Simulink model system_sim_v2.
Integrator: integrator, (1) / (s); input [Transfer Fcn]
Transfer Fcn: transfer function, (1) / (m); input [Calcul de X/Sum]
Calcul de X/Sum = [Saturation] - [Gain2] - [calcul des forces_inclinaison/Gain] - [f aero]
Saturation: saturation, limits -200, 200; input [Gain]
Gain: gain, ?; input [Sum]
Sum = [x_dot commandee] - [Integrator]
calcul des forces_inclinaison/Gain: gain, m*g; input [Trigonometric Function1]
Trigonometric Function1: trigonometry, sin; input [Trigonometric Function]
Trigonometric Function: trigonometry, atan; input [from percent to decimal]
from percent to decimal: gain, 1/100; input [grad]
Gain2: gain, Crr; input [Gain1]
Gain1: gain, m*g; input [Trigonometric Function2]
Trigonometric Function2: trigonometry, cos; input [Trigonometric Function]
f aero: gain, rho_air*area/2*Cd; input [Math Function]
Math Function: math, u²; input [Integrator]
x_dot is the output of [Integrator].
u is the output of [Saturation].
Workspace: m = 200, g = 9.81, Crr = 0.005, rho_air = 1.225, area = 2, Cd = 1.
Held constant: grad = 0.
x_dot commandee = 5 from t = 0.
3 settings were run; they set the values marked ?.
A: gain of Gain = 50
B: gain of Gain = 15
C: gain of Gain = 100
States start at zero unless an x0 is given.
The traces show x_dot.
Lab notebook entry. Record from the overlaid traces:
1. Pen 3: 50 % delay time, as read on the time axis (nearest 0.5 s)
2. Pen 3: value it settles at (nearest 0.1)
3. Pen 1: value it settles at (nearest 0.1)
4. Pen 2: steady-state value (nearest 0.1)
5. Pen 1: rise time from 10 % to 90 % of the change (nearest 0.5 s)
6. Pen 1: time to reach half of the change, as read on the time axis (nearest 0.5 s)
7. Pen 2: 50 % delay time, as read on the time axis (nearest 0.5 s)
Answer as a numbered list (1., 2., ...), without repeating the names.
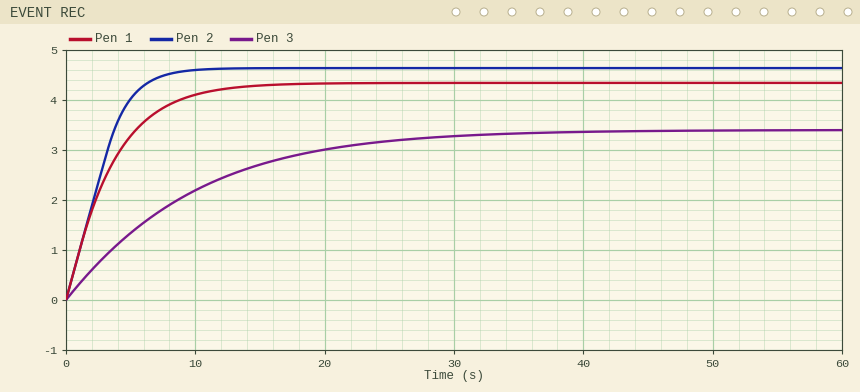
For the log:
1. 7.0 s
2. 3.4
3. 4.3
4. 4.6
5. 7.5 s
6. 2.5 s
7. 2.5 s
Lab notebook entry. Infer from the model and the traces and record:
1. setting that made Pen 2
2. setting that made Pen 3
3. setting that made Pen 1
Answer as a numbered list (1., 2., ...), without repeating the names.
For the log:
1. C
2. B
3. A
